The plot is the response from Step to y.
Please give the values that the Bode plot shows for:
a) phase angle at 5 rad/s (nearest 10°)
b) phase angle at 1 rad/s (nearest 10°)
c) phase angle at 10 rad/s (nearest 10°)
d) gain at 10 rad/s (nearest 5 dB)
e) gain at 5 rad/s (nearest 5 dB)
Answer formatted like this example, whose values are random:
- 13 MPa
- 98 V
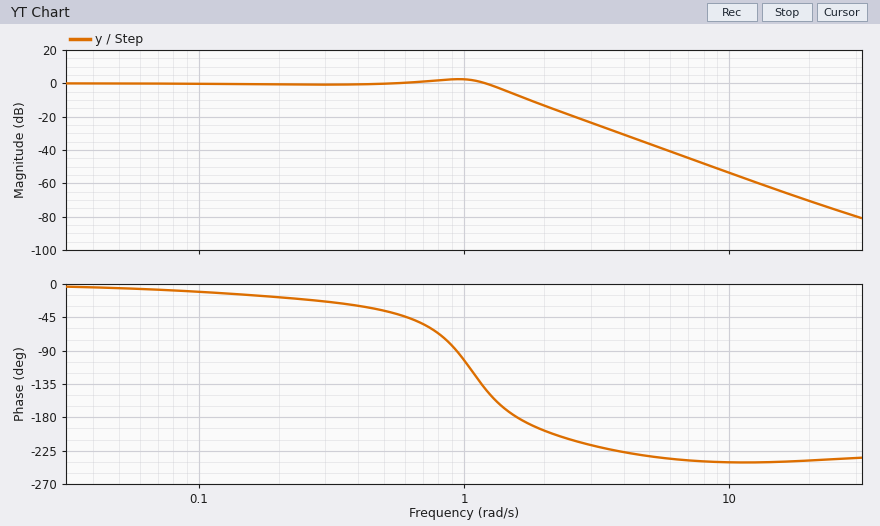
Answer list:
- -230°
- -100°
- -240°
- -55 dB
- -35 dB
